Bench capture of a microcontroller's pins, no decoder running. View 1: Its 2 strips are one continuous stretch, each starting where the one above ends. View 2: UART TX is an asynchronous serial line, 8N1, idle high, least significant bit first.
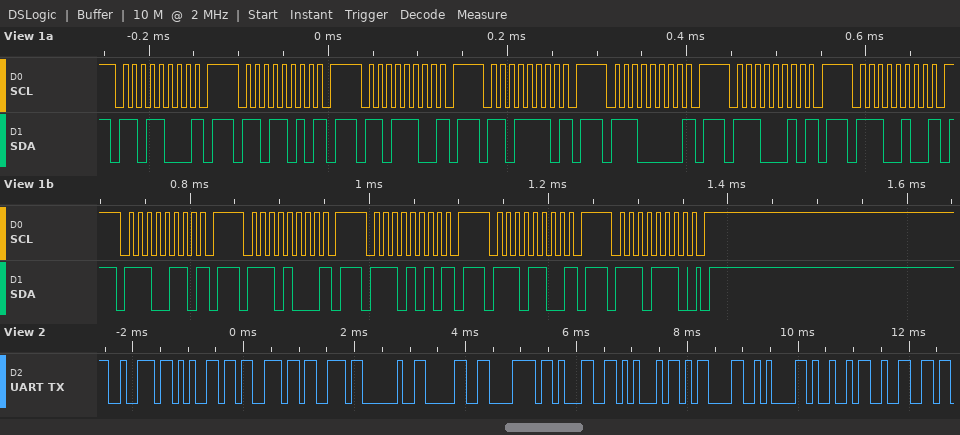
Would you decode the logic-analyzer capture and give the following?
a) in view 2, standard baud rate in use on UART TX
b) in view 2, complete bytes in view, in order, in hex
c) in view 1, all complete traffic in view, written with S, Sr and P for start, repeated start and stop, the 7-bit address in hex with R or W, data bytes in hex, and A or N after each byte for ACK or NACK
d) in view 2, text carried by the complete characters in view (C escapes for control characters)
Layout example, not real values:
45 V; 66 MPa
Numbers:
9600 baud; 72 65 73 73 20 30 78 31 45 0D 0A 49 32; S 6CW N P S 6DW N P S 6EW N P S 6FW N P S 70W N P S 71W N P S 72W N P S 73W N P S 74W N P S 75W N P S 76W N P S 77W A P; "ress 0x1E\r\nI2"
